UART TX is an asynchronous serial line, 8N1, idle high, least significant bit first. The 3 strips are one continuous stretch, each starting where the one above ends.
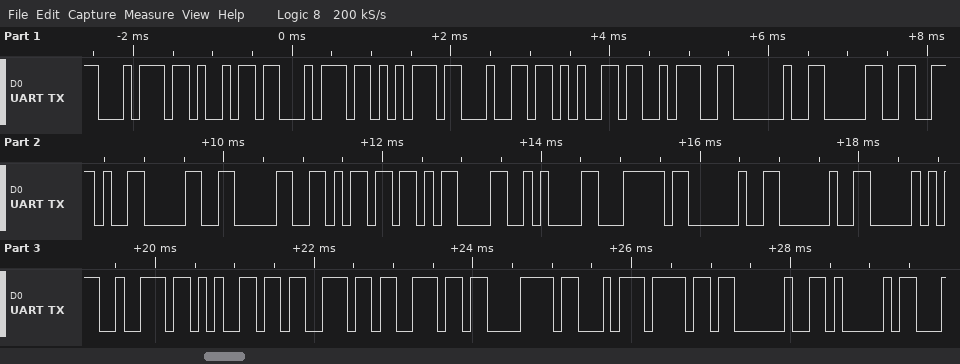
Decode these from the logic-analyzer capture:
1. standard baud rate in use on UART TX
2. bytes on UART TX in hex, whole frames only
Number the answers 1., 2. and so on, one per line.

1. 9600 baud
2. 74 69 74 75 64 65 3A 20 30 2E 30 30 6D 0D 0A 7C 20 20 50 72 65 73 73 C3 A3 6F 20 41
